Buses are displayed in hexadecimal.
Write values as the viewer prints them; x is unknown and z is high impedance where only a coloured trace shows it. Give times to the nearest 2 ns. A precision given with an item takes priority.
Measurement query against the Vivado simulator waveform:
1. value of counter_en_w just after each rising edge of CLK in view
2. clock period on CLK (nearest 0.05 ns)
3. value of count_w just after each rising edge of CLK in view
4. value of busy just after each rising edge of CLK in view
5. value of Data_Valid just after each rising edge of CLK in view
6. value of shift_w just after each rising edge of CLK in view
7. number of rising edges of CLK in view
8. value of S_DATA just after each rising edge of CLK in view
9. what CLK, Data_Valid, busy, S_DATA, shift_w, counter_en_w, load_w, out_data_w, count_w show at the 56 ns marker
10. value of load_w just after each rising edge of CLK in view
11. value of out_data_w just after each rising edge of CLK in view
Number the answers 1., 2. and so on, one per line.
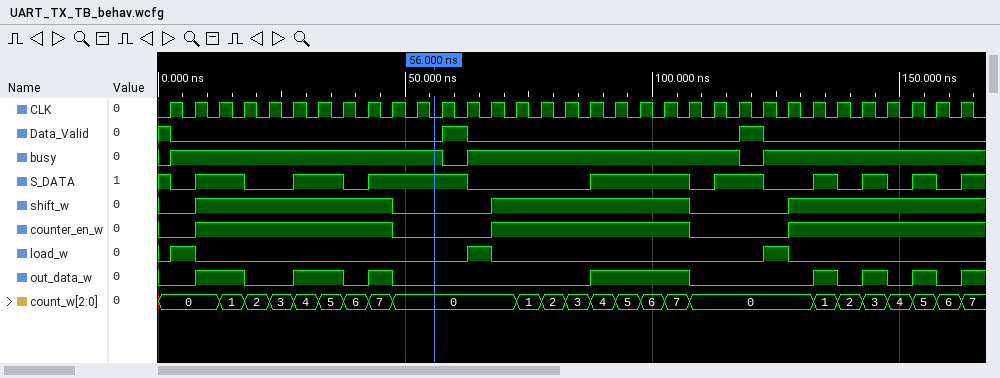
1. 0 1 1 1 1 1 1 1 1 0 0 0 0 1 1 1 1 1 1 1 1 0 0 0 0 1 1 1 1 1 1 1 1
2. 5 ns
3. 0, 0, 1, 2, 3, 4, 5, 6, 7, 0, 0, 0, 0, 0, 1, 2, 3, 4, 5, 6, 7, 0, 0, 0, 0, 0, 1, 2, 3, 4, 5, 6, 7
4. 1 1 1 1 1 1 1 1 1 1 1 0 1 1 1 1 1 1 1 1 1 1 1 0 1 1 1 1 1 1 1 1 1
5. 0 0 0 0 0 0 0 0 0 0 0 1 0 0 0 0 0 0 0 0 0 0 0 1 0 0 0 0 0 0 0 0 0
6. 0 1 1 1 1 1 1 1 1 0 0 0 0 1 1 1 1 1 1 1 1 0 0 0 0 1 1 1 1 1 1 1 1
7. 33
8. 0 1 1 0 0 1 1 0 1 1 1 1 0 0 0 0 0 1 1 1 1 0 1 1 0 0 1 0 1 0 1 0 1
9. CLK=0, Data_Valid=0, busy=1, S_DATA=1, shift_w=0, counter_en_w=0, load_w=0, out_data_w=0, count_w=0
10. 1 0 0 0 0 0 0 0 0 0 0 0 1 0 0 0 0 0 0 0 0 0 0 0 1 0 0 0 0 0 0 0 0
11. 0 1 1 0 0 1 1 0 1 0 0 0 0 0 0 0 0 1 1 1 1 0 0 0 0 0 1 0 1 0 1 0 1
